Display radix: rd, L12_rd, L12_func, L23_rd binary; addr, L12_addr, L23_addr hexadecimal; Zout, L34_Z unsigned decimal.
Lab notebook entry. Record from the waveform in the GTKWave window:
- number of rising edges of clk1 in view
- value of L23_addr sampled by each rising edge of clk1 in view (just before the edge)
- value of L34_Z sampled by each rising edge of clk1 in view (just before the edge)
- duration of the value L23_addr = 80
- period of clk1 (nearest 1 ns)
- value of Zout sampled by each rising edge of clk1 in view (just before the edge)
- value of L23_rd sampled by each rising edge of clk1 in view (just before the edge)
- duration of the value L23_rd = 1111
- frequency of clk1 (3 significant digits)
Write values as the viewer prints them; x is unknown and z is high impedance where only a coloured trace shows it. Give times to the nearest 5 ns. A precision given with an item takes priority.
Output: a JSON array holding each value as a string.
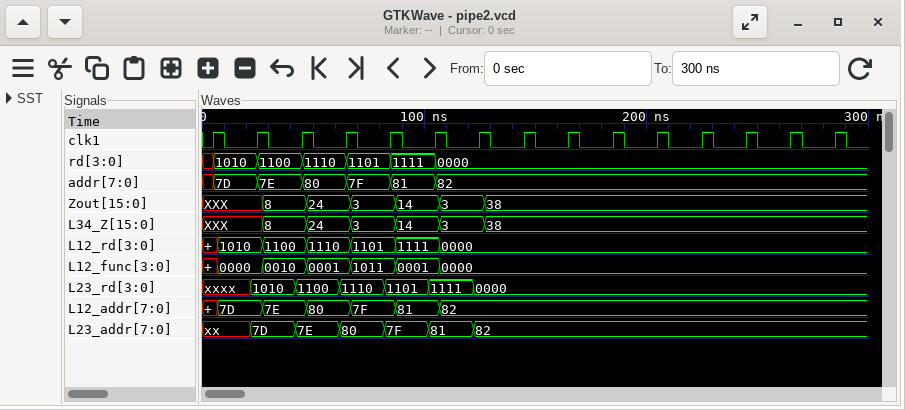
["15", "xx, 7D, 7E, 80, 7F, 81, 82, 82, 82, 82, 82, 82, 82, 82, 82", "XXX, XXX, 8, 24, 3, 14, 3, 38, 38, 38, 38, 38, 38, 38, 38", "20 ns", "20 ns", "XXX, XXX, 8, 24, 3, 14, 3, 38, 38, 38, 38, 38, 38, 38, 38", "xxxx, 1010, 1100, 1110, 1101, 1111, 0000, 0000, 0000, 0000, 0000, 0000, 0000, 0000, 0000", "20 ns", "50.0 MHz"]
